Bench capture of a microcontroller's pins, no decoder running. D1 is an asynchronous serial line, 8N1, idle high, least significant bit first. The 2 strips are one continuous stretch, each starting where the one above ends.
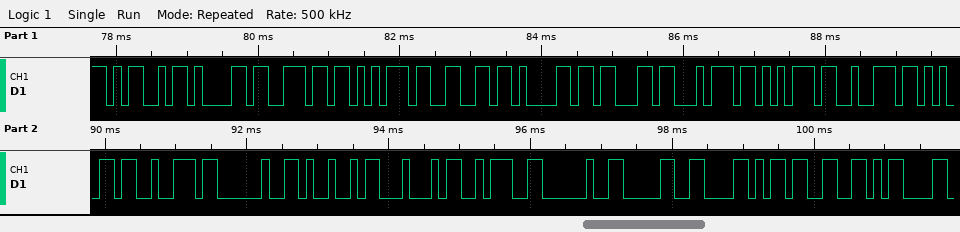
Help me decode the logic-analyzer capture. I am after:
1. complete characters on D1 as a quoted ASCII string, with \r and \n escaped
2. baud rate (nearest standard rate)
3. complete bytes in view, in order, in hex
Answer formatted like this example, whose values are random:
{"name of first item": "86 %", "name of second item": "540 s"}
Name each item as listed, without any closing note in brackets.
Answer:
{"complete characters on D1 as a quoted ASCII string, with \\r and \\n escaped": "\"Manufacturer ID: 0X3\\r\"", "baud rate": "9600 baud", "complete bytes in view, in order, in hex": "4D 61 6E 75 66 61 63 74 75 72 65 72 20 49 44 3A 20 30 58 33 0D"}
